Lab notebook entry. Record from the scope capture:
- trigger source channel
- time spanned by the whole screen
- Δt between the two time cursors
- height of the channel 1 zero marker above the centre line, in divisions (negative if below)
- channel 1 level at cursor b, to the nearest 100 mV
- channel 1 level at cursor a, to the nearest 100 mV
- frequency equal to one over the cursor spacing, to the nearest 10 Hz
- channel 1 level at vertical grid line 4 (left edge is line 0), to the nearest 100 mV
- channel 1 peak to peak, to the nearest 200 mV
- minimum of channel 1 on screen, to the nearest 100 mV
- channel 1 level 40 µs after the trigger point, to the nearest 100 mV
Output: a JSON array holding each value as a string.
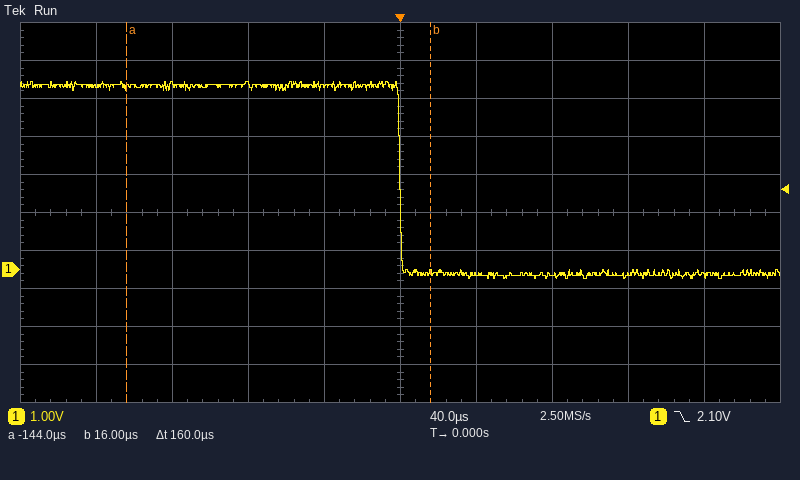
["channel 1", "400 µs", "160 µs", "-1.5 div", "-100 mV", "4.8 V", "6.25 kHz", "4.8 V", "5.2 V", "-200 mV", "-100 mV"]
